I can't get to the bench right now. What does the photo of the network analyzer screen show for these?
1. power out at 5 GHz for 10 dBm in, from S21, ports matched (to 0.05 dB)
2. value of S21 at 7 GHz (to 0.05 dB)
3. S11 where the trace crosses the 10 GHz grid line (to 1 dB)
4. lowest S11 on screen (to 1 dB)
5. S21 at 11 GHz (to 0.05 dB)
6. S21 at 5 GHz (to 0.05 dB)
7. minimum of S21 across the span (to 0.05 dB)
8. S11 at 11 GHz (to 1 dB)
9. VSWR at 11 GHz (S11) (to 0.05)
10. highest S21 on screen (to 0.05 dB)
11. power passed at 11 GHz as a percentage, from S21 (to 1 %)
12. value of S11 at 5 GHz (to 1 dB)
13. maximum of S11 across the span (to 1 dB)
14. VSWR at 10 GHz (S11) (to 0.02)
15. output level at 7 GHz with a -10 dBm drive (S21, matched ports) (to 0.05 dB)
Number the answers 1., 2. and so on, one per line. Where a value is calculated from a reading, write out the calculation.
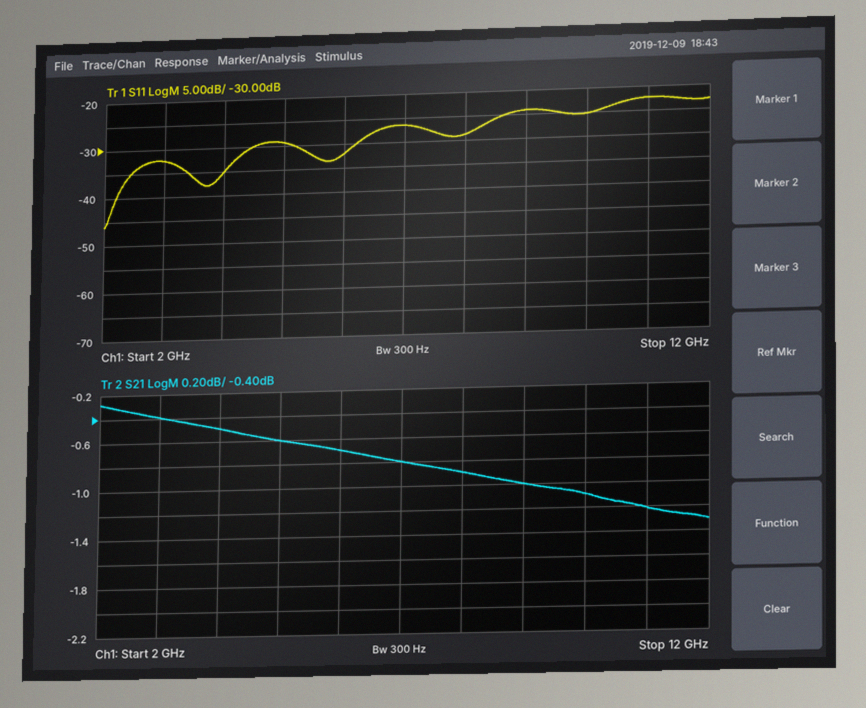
1. 10 dBm + (-0.60 dB) = 9.40 dBm
2. -0.80 dB
3. -25 dB
4. -46 dB
5. -1.20 dB
6. -0.60 dB
7. -1.30 dB
8. -22 dB
9. |Γ| = 10^(-22/20) = 0.0794; VSWR = (1 + 0.0794)/(1 − 0.0794) ≈ 1.17, so 1.15 to the nearest 0.05
10. -0.30 dB
11. 10^(-1.2/10) ≈ 76 %
12. -29 dB
13. -22 dB
14. |Γ| = 10^(-25/20) = 0.0562; VSWR = (1 + 0.0562)/(1 − 0.0562) ≈ 1.12
15. -10 dBm + (-0.80 dB) = -10.80 dBm
